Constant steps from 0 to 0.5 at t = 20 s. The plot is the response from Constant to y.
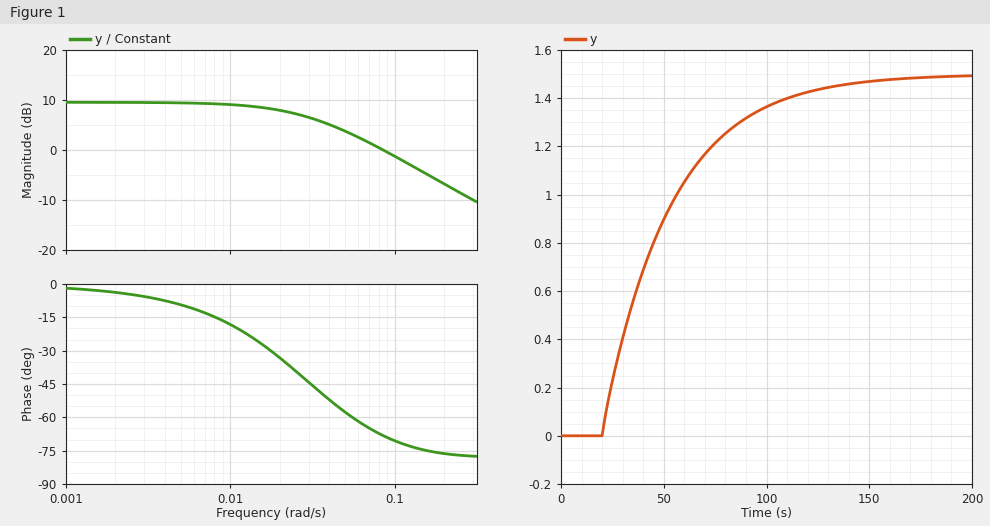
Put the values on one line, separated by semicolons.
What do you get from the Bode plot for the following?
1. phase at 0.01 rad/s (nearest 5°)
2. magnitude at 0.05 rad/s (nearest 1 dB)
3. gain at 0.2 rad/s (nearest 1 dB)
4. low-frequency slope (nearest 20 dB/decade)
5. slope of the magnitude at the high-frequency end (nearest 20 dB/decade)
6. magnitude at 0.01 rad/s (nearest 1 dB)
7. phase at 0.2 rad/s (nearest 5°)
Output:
-20°; 4 dB; -7 dB; 0 dB/decade; -20 dB/decade; 9 dB; -75°
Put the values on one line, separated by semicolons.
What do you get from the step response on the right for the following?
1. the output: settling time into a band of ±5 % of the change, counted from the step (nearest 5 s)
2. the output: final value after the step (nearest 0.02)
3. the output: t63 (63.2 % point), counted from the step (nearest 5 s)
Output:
100 s; 1.50; 35 s
